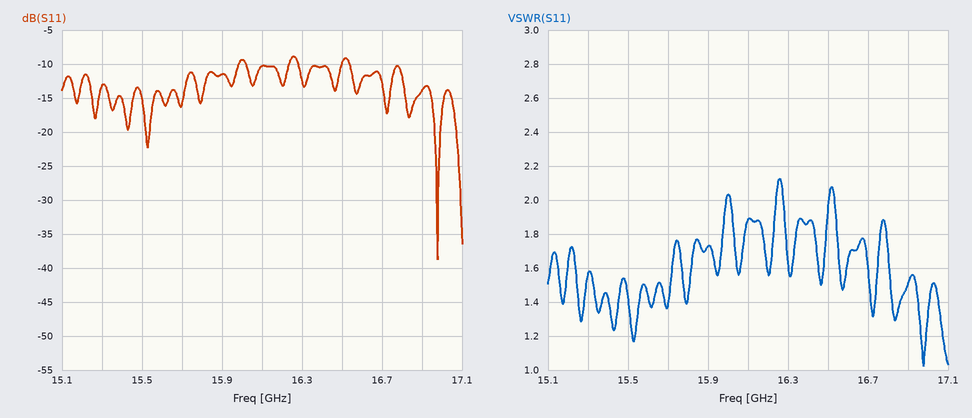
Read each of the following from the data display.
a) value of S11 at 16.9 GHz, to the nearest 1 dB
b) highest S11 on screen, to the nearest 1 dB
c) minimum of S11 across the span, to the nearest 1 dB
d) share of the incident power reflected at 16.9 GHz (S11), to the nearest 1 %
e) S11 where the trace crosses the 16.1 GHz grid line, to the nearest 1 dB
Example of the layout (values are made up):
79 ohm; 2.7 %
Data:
-14 dB; -9 dB; -39 dB; 4 %; -10 dB
